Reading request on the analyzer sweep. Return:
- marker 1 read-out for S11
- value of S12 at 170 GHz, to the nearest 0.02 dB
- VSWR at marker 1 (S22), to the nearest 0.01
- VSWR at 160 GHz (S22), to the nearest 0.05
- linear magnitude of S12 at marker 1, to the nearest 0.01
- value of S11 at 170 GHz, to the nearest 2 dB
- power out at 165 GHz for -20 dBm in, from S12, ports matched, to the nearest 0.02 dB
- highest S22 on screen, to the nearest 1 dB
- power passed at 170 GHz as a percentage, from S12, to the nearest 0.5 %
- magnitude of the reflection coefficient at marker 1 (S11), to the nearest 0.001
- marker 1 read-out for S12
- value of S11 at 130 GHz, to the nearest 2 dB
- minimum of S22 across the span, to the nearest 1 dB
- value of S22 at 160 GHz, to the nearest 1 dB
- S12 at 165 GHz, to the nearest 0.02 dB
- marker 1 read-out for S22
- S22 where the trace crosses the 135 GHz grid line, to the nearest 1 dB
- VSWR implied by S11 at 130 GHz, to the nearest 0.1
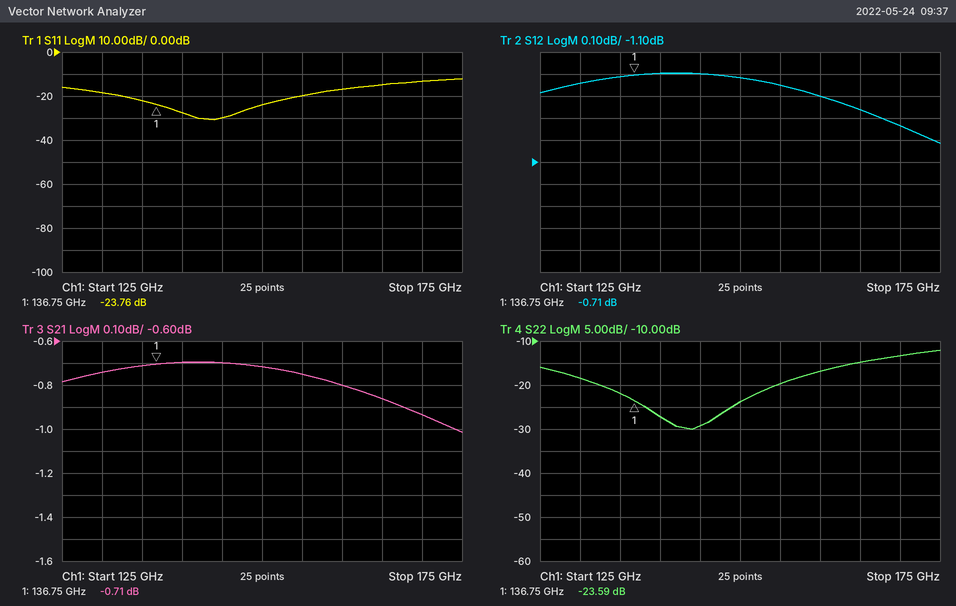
-23.76 dB
-0.94 dB
1.14
1.35
0.92
-14 dB
-20.86 dBm
-12 dB
80.5 %
0.065
-0.71 dB
-18 dB
-30 dB
-17 dB
-0.86 dB
-23.59 dB
-22 dB
1.3
